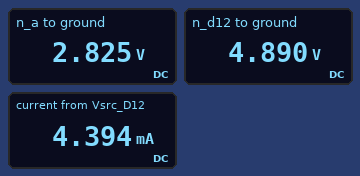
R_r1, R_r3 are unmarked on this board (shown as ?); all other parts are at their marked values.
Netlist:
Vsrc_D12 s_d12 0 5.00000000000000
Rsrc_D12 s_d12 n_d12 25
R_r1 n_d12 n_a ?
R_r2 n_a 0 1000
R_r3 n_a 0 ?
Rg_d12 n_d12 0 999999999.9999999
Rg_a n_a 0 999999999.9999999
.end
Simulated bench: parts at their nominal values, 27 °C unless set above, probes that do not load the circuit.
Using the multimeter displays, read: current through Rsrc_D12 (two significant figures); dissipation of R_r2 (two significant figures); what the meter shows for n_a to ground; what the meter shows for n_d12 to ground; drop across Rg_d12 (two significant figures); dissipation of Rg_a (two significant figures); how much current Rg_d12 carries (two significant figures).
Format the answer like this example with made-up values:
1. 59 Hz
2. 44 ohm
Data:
1. 4.4 mA
2. 8.0 mW
3. 2.825 V
4. 4.890 V
5. 4.9 V
6. 8.0 nW
7. 4.9 nA
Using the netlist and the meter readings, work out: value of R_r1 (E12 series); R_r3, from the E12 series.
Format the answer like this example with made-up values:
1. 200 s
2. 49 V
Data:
1. 470 Ω
2. 1.8 kΩ
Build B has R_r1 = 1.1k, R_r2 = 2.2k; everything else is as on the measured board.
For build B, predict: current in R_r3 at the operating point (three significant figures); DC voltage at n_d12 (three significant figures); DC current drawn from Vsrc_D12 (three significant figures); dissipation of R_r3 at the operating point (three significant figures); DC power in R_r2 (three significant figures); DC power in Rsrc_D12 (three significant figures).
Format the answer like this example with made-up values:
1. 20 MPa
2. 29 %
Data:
1. 1.30 mA
2. 4.94 V
3. 2.36 mA
4. 3.04 mW
5. 2.49 mW
6. 140 µW
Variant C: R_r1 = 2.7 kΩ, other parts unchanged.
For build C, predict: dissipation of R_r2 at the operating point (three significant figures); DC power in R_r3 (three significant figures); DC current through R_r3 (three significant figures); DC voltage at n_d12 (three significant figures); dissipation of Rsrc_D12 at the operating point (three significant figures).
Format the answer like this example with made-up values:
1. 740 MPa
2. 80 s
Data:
1. 911 µW
2. 506 µW
3. 530 µA
4. 4.96 V
5. 55.1 µW
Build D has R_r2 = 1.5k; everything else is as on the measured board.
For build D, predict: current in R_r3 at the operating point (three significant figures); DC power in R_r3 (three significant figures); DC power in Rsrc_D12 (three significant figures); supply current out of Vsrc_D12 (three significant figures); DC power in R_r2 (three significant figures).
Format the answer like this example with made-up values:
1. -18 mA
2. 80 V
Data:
1. 1.73 mA
2. 5.39 mW
3. 362 µW
4. 3.81 mA
5. 6.47 mW
